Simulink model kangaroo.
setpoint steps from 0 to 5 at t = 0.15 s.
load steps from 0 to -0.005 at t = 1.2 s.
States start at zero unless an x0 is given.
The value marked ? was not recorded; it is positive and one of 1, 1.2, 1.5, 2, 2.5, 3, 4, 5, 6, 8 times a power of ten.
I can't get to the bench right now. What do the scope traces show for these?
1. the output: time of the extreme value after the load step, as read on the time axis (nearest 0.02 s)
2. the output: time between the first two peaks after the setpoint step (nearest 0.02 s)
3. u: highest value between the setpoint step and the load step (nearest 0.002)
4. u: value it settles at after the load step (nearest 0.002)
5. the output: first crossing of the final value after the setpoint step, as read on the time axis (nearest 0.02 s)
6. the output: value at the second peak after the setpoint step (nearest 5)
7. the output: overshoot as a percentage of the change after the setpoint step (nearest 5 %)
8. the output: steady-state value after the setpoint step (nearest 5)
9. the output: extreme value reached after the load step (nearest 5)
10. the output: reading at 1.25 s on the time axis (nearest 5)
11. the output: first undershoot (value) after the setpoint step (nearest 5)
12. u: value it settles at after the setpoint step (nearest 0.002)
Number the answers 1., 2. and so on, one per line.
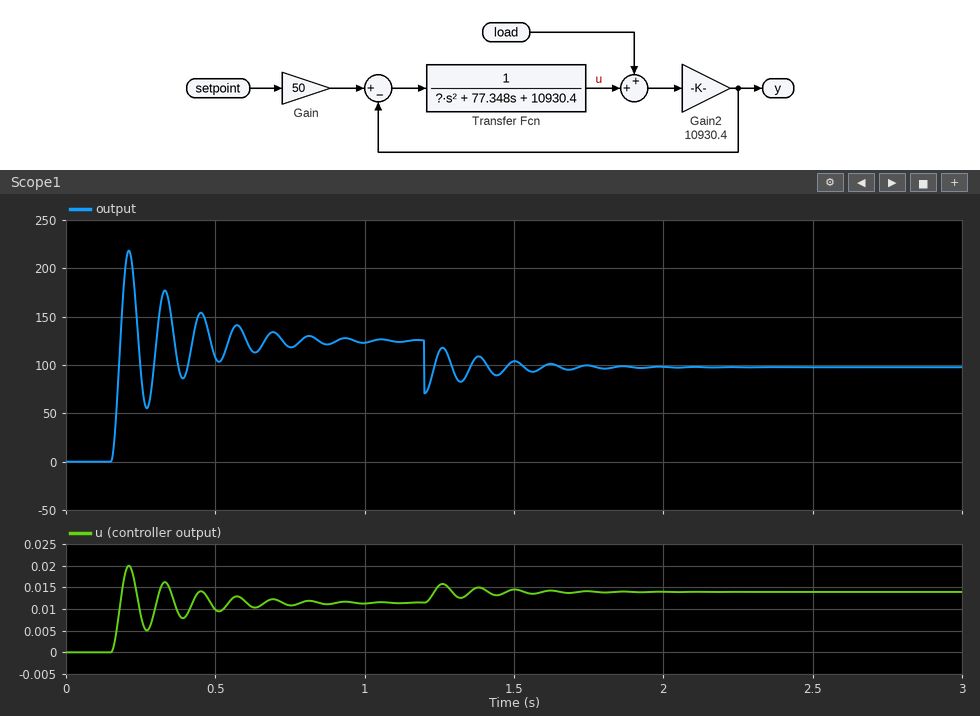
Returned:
1. 1.20 s
2. 0.12 s
3. 0.020
4. 0.014
5. 0.18 s
6. 175
7. 75 %
8. 125
9. 70
10. 115
11. 55
12. 0.012
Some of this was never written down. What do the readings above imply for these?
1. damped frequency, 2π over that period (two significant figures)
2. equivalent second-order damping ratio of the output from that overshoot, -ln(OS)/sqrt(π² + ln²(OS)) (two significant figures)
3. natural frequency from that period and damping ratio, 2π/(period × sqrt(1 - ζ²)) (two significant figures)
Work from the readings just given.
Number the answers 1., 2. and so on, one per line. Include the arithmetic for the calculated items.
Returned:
1. 2π / 0.12 = 52 rad/s
2. ln(0.75) = -0.288; 0.288 / sqrt(9.870 + 0.083) = 0.091
3. 2π / (0.12 × sqrt(1 - 0.091²)) = 53 rad/s
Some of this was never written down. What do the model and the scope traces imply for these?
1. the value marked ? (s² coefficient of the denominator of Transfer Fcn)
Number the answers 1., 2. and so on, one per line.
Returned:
1. 8
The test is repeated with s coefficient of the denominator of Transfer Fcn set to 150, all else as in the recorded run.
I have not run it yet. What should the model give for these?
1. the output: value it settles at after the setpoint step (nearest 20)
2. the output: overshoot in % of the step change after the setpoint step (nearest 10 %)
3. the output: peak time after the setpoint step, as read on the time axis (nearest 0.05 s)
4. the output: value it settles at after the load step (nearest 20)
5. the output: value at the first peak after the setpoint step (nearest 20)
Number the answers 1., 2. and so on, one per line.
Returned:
1. 120
2. 60 %
3. 0.20 s
4. 100
5. 200
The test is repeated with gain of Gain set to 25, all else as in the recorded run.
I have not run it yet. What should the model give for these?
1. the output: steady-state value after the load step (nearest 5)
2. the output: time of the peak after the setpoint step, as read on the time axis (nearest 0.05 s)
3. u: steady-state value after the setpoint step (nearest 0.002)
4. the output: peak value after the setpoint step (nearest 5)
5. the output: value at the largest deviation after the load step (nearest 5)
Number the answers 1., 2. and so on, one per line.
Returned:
1. 35
2. 0.20 s
3. 0.006
4. 110
5. 10
